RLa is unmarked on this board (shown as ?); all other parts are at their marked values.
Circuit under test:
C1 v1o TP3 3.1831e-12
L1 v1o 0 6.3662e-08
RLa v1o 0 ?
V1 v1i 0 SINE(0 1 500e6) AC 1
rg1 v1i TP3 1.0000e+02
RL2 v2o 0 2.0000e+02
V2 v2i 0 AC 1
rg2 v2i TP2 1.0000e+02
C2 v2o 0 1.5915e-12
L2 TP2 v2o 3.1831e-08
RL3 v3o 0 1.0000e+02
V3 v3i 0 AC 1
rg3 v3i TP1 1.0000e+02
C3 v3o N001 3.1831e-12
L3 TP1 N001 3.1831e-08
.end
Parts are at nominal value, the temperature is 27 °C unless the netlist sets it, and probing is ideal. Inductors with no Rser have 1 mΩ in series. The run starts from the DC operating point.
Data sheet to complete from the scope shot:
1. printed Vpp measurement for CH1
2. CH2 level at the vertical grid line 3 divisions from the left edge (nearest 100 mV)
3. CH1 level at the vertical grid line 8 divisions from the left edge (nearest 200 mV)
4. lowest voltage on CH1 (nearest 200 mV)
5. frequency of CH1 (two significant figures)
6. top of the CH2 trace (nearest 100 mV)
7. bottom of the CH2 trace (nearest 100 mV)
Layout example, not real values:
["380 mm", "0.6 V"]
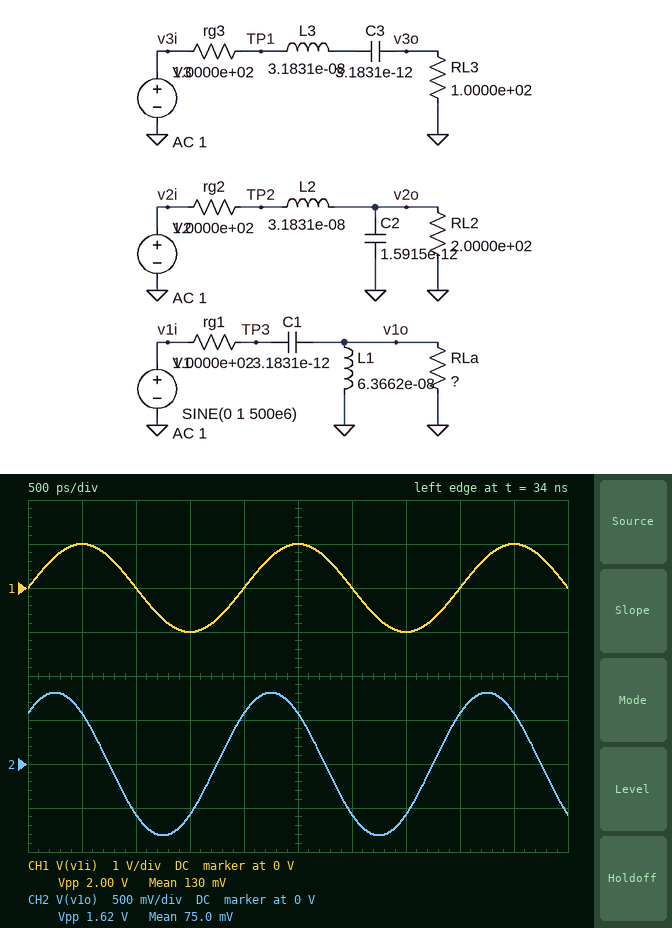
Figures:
["2.00 V", "-600 mV", "0 V", "-1.0 V", "500 MHz", "800 mV", "-800 mV"]
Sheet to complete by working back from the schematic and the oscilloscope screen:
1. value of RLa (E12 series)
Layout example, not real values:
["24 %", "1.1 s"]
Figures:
["270 Ω"]
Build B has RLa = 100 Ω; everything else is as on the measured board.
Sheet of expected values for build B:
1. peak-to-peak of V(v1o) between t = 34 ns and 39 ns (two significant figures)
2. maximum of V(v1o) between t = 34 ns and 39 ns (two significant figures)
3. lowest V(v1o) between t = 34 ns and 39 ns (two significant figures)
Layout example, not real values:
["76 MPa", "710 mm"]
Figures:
["940 mV", "470 mV", "-470 mV"]
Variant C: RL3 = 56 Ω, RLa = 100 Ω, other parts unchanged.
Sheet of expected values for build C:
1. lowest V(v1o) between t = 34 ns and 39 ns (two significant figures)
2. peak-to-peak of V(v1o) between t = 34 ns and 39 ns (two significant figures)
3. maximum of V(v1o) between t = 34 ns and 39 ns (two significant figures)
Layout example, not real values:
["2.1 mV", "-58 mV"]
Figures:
["-470 mV", "940 mV", "470 mV"]
